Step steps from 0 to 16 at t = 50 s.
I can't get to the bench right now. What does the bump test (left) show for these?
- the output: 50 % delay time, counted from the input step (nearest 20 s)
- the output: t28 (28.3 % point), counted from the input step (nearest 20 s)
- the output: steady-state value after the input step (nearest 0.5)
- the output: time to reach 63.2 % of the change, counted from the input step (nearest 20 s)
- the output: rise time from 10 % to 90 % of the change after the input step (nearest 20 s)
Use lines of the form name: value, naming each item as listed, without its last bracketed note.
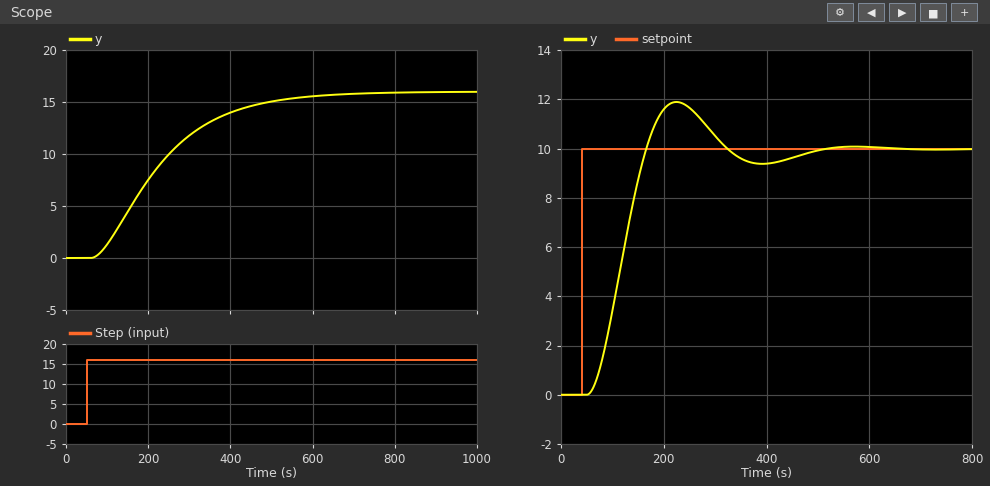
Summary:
the output: 50 % delay time, counted from the input step: 160 s
the output: t28 (28.3 % point), counted from the input step: 100 s
the output: steady-state value after the input step: 16.0
the output: time to reach 63.2 % of the change, counted from the input step: 200 s
the output: rise time from 10 % to 90 % of the change after the input step: 320 s
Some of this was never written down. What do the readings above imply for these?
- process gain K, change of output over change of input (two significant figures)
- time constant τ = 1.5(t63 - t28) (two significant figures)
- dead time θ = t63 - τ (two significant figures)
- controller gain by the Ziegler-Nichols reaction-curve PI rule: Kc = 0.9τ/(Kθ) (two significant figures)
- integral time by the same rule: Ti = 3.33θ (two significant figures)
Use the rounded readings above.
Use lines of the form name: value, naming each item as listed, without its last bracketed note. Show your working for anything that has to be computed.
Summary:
process gain K, change of output over change of input: (16 - 0) / 16 = 1.0
time constant τ = 1.5(t63 - t28): 1.5 × (200 - 100) = 150 s
dead time θ = t63 - τ: 200 - 150 = 50 s
controller gain by the Ziegler-Nichols reaction-curve PI rule: Kc = 0.9τ/(Kθ): 0.9 × 150 / (1 × 50) = 2.7
integral time by the same rule: Ti = 3.33θ: 3.33 × 50 = 170 s
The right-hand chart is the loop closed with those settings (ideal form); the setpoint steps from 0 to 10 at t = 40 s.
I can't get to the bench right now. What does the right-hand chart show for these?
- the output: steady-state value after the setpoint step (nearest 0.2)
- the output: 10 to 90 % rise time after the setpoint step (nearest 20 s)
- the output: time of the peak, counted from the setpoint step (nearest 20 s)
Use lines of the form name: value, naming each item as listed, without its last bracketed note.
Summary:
the output: steady-state value after the setpoint step: 10.0
the output: 10 to 90 % rise time after the setpoint step: 80 s
the output: time of the peak, counted from the setpoint step: 180 s
